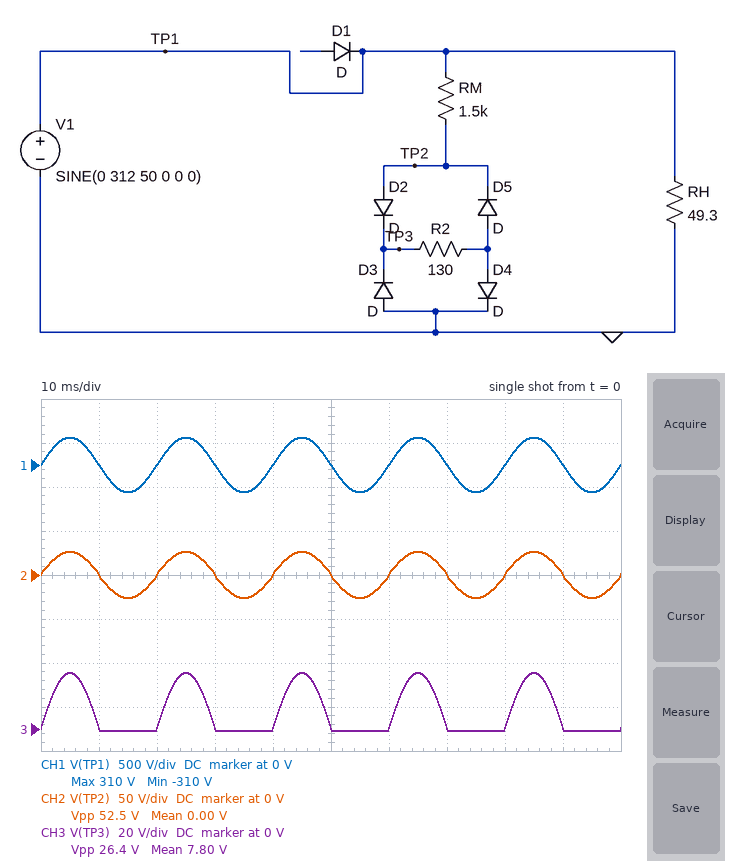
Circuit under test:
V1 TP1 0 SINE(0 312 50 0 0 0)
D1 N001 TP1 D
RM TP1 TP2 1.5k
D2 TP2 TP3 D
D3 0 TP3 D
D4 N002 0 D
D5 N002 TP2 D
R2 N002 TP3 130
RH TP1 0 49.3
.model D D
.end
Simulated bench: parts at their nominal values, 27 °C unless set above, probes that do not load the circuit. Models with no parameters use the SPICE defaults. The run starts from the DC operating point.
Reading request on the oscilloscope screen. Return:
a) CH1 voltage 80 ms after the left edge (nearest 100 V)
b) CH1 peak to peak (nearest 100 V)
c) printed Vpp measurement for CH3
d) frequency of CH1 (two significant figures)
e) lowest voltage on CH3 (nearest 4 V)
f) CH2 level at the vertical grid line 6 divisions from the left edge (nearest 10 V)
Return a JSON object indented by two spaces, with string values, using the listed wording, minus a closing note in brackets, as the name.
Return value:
{
  "CH1 voltage 80 ms after the left edge": "0 V",
  "CH1 peak to peak": "600 V",
  "printed Vpp measurement for CH3": "26.4 V",
  "frequency of CH1": "50 Hz",
  "lowest voltage on CH3": "0 V",
  "CH2 level at the vertical grid line 6 divisions from the left edge": "0 V"
}
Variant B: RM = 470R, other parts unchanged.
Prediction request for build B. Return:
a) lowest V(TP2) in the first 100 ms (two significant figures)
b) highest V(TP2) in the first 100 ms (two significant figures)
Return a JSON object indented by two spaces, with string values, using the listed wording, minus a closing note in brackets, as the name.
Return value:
{
  "lowest V(TP2) in the first 100 ms": "-69 V",
  "highest V(TP2) in the first 100 ms": "69 V"
}
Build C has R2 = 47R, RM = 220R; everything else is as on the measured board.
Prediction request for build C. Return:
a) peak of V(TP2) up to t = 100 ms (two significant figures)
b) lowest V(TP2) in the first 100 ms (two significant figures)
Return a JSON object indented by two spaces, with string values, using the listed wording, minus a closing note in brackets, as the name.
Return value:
{
  "peak of V(TP2) up to t = 100 ms": "56 V",
  "lowest V(TP2) in the first 100 ms": "-56 V"
}
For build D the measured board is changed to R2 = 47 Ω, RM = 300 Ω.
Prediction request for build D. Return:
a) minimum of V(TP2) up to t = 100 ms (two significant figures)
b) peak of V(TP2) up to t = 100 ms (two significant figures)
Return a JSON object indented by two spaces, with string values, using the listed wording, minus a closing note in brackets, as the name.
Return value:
{
  "minimum of V(TP2) up to t = 100 ms": "-44 V",
  "peak of V(TP2) up to t = 100 ms": "44 V"
}
